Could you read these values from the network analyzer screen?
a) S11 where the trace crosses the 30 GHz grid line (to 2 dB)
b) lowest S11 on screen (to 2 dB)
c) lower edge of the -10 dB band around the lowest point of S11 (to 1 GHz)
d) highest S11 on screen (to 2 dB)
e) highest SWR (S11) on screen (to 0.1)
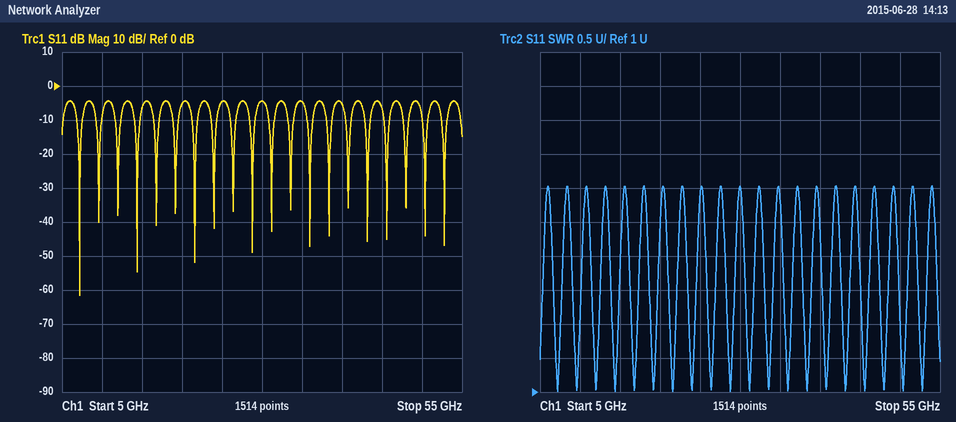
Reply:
-4 dB
-62 dB
7 GHz
-4 dB
4.0
